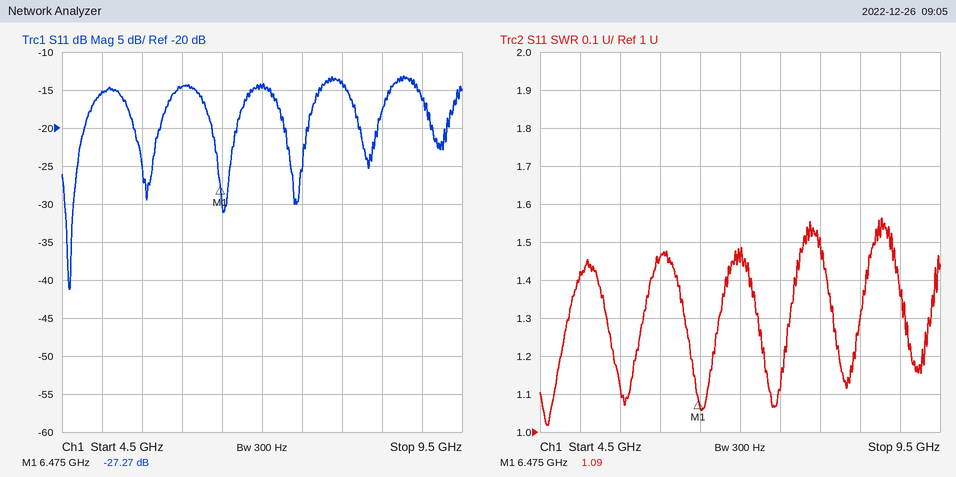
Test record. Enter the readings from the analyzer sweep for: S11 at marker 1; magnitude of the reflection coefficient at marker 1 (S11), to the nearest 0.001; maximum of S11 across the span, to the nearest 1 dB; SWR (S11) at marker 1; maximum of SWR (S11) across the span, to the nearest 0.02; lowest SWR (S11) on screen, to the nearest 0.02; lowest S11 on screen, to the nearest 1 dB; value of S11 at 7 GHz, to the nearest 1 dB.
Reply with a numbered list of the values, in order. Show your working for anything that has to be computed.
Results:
1. -27.27 dB
2. 10^(-27.27/20) ≈ 0.043
3. -13 dB
4. 1.09
5. 1.56
6. 1.02
7. -41 dB
8. -15 dB
